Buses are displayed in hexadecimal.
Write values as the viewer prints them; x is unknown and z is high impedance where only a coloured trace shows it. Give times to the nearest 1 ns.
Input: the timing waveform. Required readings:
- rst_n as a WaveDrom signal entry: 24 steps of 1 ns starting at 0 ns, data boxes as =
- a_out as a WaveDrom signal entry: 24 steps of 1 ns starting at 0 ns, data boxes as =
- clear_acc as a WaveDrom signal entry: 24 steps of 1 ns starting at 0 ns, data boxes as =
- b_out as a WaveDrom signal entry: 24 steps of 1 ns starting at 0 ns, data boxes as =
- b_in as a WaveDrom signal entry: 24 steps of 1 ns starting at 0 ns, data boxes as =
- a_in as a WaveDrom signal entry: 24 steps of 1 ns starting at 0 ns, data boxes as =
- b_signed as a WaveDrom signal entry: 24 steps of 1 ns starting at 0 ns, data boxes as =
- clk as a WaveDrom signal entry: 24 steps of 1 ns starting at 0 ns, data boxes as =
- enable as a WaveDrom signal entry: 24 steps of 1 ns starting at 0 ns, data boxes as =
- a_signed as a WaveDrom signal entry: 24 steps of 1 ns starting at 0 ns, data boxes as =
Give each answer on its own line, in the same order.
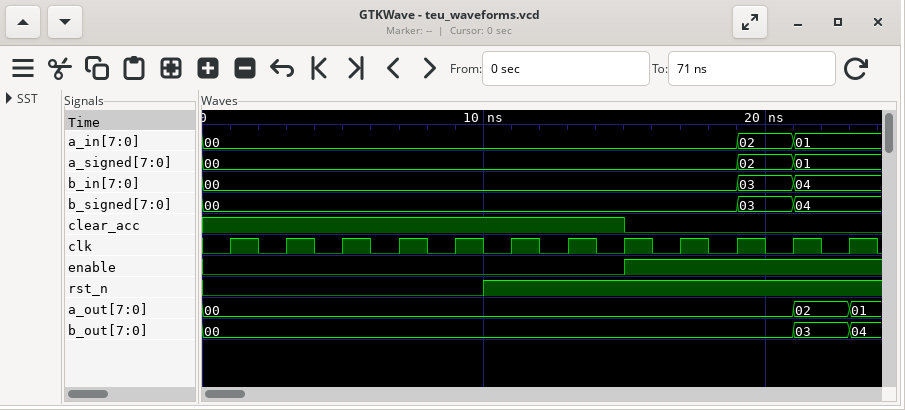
{name: 'rst_n', wave: '0.........1.............'}
{name: 'a_out', wave: '=....................=.=', data: '00 02 01'}
{name: 'clear_acc', wave: '1..............0........'}
{name: 'b_out', wave: '=....................=.=', data: '00 03 04'}
{name: 'b_in', wave: '=..................=.=..', data: '00 03 04'}
{name: 'a_in', wave: '=..................=.=..', data: '00 02 01'}
{name: 'b_signed', wave: '=..................=.=..', data: '00 03 04'}
{name: 'clk', wave: '010101010101010101010101'}
{name: 'enable', wave: '0..............1........'}
{name: 'a_signed', wave: '=..................=.=..', data: '00 02 01'}
